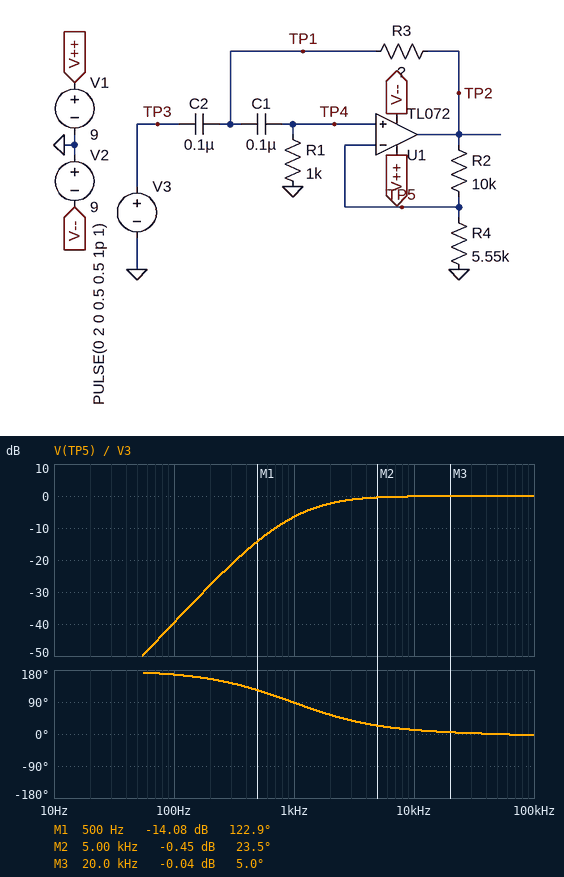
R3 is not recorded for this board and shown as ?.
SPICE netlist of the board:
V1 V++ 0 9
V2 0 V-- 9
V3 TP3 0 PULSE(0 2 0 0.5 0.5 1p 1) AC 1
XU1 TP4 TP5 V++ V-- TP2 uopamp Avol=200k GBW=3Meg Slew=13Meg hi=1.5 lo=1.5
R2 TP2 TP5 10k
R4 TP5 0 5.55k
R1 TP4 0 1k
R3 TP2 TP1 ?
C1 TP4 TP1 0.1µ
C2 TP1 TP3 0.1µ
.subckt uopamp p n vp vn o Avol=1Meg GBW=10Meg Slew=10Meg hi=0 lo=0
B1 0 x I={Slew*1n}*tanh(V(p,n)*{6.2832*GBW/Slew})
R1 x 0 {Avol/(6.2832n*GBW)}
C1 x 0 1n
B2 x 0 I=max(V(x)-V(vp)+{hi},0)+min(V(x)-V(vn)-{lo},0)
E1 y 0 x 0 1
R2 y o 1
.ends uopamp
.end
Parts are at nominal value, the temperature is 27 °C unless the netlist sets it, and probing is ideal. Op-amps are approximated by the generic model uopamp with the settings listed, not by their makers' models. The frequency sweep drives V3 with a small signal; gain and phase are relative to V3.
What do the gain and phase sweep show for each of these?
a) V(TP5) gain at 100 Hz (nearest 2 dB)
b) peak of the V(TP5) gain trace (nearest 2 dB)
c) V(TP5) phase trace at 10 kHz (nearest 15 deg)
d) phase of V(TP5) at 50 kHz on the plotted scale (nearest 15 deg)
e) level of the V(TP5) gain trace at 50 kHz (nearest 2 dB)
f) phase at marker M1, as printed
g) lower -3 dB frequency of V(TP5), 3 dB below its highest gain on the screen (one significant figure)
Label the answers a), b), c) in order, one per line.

a) -40 dB
b) 0 dB
c) 15 deg
d) 0 deg
e) 0 dB
f) 122.9 deg
g) 2 kHz
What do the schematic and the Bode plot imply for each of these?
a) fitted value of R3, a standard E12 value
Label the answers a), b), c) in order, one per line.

a) 2.7 kΩ
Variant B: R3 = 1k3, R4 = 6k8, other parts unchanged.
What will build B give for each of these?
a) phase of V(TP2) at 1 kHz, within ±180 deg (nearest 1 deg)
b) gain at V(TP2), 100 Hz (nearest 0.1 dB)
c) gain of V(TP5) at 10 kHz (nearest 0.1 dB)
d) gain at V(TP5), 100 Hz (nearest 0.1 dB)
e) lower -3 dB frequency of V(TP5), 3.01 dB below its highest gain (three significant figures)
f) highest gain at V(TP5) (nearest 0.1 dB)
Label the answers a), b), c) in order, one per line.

a) 124 deg
b) -37.9 dB
c) 0.1 dB
d) -45.8 dB
e) 1.19 kHz
f) 1.3 dB
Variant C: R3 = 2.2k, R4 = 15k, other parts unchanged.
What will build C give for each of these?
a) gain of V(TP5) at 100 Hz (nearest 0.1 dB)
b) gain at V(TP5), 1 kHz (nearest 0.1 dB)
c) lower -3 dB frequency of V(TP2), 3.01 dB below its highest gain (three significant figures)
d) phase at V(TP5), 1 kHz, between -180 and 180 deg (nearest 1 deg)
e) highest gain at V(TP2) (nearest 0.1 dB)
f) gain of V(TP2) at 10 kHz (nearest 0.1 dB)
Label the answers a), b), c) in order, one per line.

a) -41.4 dB
b) -8.6 dB
c) 2.28 kHz
d) 93 deg
e) 4.4 dB
f) 4.2 dB
